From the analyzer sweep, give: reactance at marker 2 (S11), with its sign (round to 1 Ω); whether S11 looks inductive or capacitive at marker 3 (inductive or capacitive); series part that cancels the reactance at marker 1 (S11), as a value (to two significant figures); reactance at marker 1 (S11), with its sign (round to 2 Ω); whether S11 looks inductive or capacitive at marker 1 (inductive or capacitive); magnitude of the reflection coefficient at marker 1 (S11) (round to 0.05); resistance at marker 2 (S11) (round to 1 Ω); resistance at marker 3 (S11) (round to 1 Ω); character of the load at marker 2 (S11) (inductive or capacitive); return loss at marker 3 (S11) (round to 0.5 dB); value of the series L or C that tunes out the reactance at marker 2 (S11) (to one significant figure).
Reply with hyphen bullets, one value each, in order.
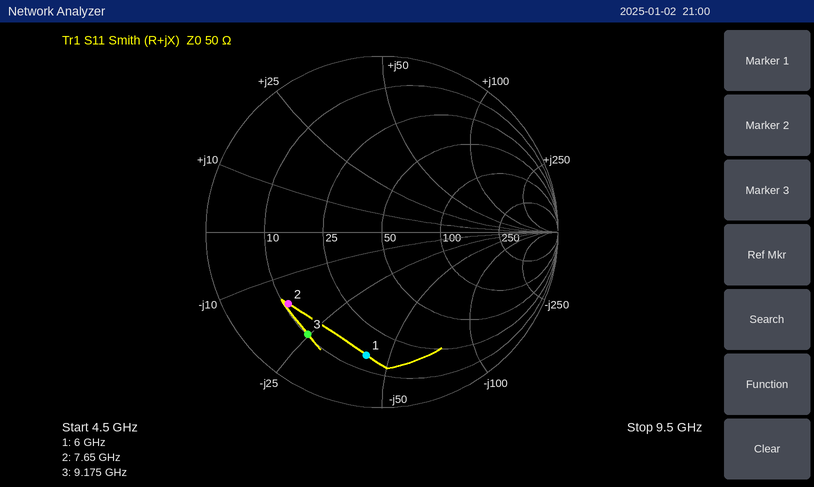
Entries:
- -16 Ω
- capacitive
- 1.1 nH
- -42 Ω
- capacitive
- 0.70
- 11 Ω
- 10 Ω
- capacitive
- 3.0 dB
- 300 pH
